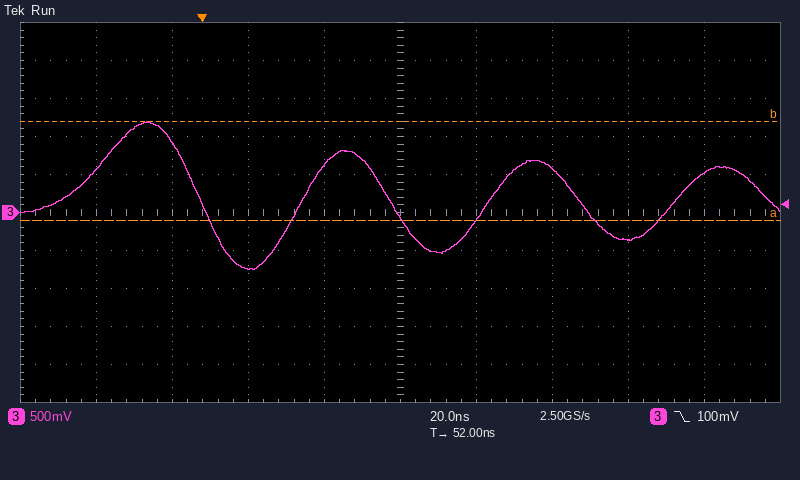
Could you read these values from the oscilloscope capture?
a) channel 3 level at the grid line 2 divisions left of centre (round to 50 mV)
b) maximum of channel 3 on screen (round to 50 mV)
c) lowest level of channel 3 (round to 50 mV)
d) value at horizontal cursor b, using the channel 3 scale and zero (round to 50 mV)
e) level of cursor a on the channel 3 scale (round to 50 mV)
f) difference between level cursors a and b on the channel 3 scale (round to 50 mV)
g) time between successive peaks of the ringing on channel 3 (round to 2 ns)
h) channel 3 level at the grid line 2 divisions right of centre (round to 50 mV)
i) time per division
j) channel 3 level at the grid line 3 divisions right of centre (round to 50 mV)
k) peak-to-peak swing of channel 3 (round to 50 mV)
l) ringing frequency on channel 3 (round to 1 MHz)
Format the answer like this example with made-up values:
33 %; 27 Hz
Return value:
-750 mV; 1.20 V; -750 mV; 1.20 V; -100 mV; 1.30 V; 50 ns; 600 mV; 20 ns; -350 mV; 1.95 V; 20 MHz
